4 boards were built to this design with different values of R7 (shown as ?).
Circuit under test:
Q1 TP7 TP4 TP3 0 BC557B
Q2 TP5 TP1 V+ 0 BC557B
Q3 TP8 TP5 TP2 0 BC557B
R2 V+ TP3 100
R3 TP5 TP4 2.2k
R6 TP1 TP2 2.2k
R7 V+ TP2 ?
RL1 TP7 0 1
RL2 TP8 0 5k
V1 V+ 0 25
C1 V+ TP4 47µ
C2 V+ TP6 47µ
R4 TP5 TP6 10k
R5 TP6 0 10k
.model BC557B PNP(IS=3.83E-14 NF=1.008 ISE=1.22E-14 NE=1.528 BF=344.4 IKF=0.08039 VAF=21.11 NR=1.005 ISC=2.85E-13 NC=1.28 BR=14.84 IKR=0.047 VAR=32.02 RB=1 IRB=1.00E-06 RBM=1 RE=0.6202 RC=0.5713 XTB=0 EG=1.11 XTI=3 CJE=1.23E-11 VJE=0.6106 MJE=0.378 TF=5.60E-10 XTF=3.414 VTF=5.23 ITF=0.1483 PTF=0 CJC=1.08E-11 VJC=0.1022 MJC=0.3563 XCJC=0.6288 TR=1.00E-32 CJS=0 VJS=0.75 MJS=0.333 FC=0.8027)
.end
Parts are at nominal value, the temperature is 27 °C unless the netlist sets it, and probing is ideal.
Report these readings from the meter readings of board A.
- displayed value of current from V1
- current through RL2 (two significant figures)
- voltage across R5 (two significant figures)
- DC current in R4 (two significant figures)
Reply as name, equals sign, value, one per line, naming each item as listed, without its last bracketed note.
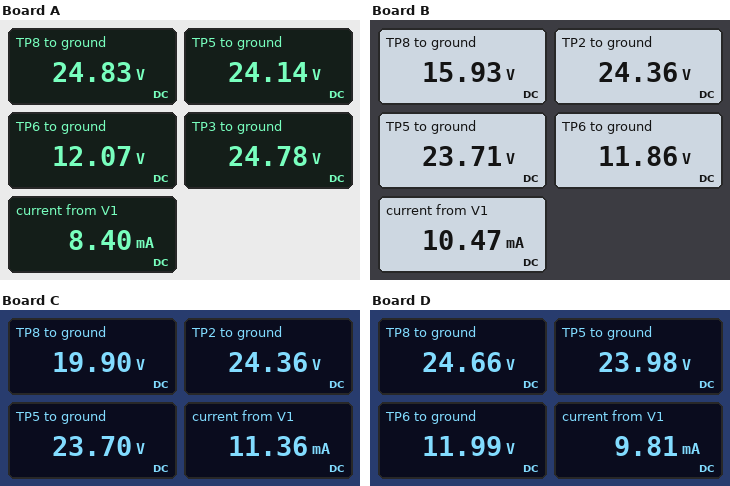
displayed value of current from V1 = 8.40 mA
current through RL2 = 5.0 mA
voltage across R5 = 12 V
DC current in R4 = 1.2 mA
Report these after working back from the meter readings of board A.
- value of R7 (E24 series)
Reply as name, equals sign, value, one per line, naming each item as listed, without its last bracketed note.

value of R7 = 24 Ω
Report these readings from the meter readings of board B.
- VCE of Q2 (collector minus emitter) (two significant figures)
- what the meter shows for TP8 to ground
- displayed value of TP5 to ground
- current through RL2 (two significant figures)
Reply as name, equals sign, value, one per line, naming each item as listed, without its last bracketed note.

VCE of Q2 (collector minus emitter) = -1.3 V
what the meter shows for TP8 to ground = 15.93 V
displayed value of TP5 to ground = 23.71 V
current through RL2 = 3.2 mA
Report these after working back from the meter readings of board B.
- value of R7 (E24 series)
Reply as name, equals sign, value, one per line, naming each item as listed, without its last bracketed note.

value of R7 = 200 Ω
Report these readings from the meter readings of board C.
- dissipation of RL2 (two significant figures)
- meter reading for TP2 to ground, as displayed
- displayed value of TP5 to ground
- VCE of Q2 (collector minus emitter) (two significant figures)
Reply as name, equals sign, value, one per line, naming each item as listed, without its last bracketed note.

dissipation of RL2 = 79 mW
meter reading for TP2 to ground, as displayed = 24.36 V
displayed value of TP5 to ground = 23.70 V
VCE of Q2 (collector minus emitter) = -1.3 V
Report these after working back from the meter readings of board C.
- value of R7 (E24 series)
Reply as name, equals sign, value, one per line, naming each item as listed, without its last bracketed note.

value of R7 = 160 Ω
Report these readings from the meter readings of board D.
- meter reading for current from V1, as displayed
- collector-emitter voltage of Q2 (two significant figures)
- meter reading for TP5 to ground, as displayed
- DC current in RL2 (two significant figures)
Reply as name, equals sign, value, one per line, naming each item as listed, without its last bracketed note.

meter reading for current from V1, as displayed = 9.81 mA
collector-emitter voltage of Q2 = -1.0 V
meter reading for TP5 to ground, as displayed = 23.98 V
DC current in RL2 = 4.9 mA
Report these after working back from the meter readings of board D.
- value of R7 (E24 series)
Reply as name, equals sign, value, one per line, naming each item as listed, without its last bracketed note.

value of R7 = 51 Ω
